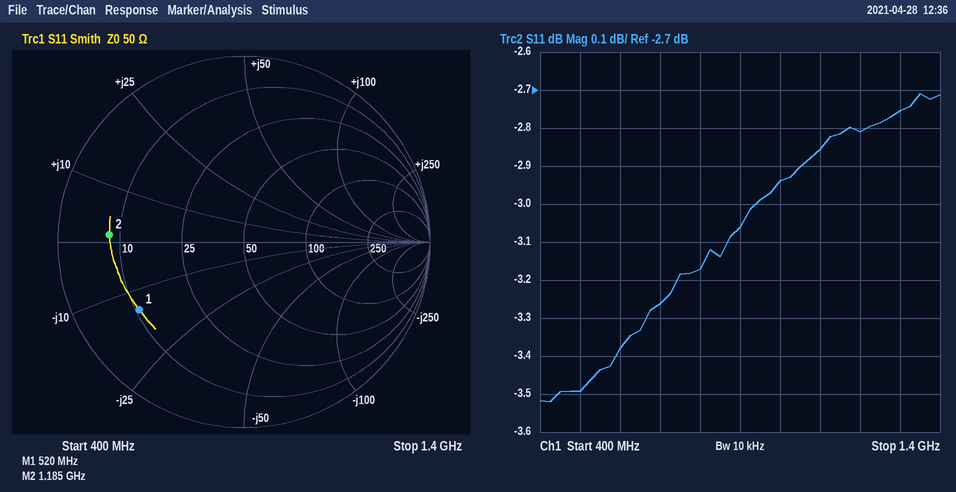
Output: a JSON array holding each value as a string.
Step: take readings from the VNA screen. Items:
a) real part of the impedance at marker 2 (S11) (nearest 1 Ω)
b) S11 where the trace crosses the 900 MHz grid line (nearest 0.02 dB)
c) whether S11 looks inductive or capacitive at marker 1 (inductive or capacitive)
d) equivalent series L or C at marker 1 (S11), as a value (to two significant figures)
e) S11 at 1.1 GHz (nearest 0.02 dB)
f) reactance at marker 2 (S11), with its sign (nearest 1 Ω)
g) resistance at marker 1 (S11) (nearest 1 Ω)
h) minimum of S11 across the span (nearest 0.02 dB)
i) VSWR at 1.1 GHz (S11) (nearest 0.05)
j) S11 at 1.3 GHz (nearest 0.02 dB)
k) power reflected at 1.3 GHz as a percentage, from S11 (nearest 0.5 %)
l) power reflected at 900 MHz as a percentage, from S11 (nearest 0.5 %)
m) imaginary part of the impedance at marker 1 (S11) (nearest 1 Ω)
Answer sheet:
["8 Ω", "-3.06 dB", "capacitive", "22 pF", "-2.86 dB", "+1 Ω", "11 Ω", "-3.52 dB", "6.15", "-2.76 dB", "53.0 %", "49.5 %", "-14 Ω"]
